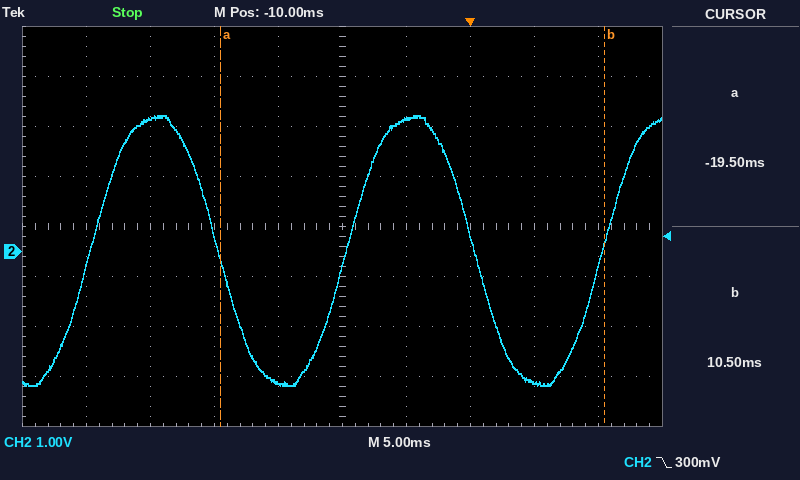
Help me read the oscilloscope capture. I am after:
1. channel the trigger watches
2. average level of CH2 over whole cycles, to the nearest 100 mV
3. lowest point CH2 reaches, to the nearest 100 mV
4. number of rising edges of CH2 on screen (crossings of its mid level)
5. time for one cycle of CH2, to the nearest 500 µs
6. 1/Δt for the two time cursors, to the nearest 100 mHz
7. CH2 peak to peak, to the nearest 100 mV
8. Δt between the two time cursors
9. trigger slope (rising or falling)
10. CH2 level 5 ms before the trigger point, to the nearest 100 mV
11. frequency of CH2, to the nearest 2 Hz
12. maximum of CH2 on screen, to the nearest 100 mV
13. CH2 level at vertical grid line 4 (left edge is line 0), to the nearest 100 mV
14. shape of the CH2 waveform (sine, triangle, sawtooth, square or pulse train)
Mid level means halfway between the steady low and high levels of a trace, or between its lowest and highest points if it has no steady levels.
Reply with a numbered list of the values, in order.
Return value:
1. CH2
2. 0.0 V
3. -2.7 V
4. 3
5. 20.0 ms
6. 33.3 Hz
7. 5.4 V
8. 30.0 ms
9. falling
10. 2.6 V
11. 50 Hz
12. 2.7 V
13. -2.6 V
14. sine
